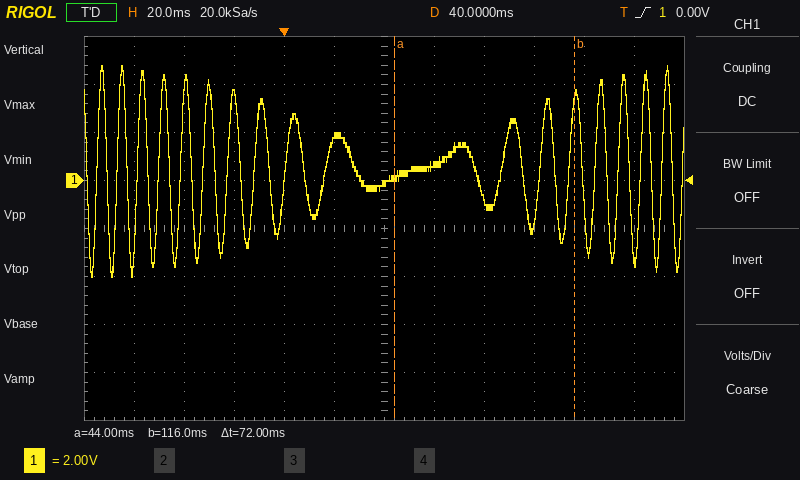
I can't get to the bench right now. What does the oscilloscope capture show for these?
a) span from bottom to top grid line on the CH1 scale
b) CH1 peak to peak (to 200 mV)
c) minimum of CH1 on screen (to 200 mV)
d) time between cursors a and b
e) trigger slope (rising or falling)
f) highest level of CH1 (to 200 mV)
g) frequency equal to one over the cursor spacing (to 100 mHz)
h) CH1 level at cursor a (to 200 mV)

16 V
8.8 V
-4.0 V
72 ms
rising
4.8 V
13.9 Hz
200 mV
